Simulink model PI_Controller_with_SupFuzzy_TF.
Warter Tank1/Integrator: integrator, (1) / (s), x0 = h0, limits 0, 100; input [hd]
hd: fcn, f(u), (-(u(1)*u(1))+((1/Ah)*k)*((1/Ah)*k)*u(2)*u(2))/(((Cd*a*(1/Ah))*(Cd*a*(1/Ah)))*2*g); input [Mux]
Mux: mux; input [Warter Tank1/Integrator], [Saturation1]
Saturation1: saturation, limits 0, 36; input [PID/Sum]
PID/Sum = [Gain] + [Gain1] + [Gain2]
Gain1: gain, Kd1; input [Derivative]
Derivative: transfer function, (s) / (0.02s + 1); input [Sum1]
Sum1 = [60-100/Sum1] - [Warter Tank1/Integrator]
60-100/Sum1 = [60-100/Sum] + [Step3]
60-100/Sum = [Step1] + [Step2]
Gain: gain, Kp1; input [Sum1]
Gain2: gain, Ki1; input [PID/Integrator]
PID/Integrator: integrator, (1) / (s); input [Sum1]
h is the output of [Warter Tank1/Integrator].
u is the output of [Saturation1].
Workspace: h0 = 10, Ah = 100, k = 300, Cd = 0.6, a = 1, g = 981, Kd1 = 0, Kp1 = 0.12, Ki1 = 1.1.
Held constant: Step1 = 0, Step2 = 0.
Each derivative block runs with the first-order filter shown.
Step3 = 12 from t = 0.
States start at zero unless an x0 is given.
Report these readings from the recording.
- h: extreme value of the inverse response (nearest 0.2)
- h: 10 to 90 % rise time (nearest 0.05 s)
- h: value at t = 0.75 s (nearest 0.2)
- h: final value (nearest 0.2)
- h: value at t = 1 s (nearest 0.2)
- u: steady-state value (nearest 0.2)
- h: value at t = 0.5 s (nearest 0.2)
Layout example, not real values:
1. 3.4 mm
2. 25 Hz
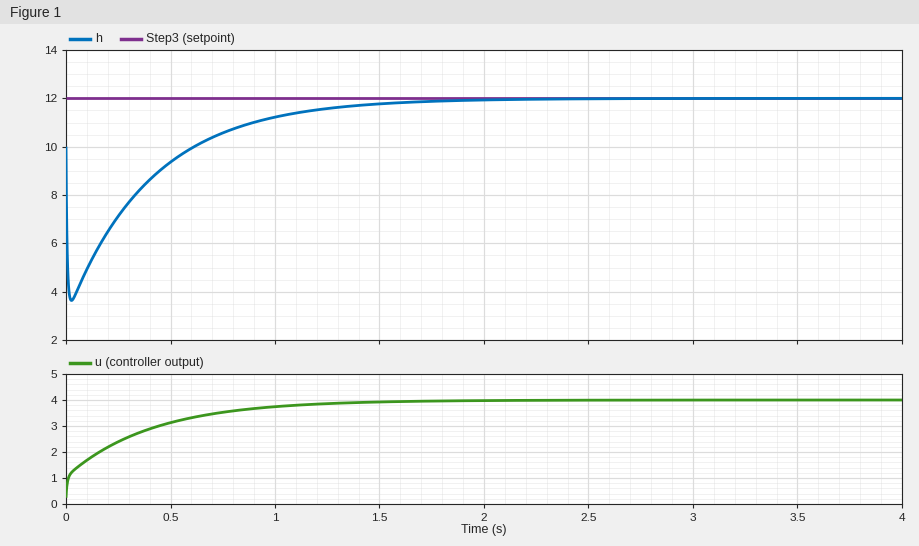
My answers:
1. 3.6
2. 0.90 s
3. 10.6
4. 12.0
5. 11.2
6. 4.0
7. 9.4
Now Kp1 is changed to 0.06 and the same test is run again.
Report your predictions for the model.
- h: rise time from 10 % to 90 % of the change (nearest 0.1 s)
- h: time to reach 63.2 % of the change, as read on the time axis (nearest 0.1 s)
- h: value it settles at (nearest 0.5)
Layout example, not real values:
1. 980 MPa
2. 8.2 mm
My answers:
1. 0.8 s
2. 0.9 s
3. 12.0
